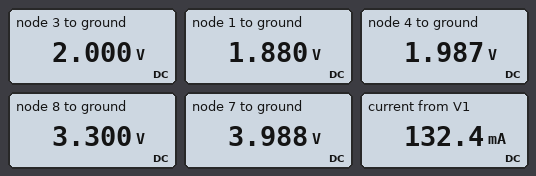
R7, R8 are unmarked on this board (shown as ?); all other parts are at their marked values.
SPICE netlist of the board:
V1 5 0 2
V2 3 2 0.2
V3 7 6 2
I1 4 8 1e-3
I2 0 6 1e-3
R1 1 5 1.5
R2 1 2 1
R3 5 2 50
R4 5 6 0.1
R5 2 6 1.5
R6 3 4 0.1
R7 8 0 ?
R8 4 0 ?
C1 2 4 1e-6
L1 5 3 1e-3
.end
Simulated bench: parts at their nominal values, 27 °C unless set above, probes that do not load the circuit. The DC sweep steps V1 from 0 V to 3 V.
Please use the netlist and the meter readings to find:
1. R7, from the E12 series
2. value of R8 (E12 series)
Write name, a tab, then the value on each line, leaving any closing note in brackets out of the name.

R7, from the E12 series	3.3 kΩ
value of R8	15 Ω
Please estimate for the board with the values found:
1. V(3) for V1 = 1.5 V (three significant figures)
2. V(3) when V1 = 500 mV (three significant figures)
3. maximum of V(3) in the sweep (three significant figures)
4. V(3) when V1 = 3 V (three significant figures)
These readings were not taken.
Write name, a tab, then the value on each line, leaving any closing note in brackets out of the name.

V(3) for V1 = 1.5 V	1.50 V
V(3) when V1 = 500 mV	500 mV
maximum of V(3) in the sweep	3.00 V
V(3) when V1 = 3 V	3.00 V
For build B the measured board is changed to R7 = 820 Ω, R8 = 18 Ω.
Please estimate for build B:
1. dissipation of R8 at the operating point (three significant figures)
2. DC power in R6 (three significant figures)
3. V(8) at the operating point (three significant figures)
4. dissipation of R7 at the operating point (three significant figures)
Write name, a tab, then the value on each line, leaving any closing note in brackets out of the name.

dissipation of R8 at the operating point	220 mW
DC power in R6	1.24 mW
V(8) at the operating point	820 mV
dissipation of R7 at the operating point	820 µW
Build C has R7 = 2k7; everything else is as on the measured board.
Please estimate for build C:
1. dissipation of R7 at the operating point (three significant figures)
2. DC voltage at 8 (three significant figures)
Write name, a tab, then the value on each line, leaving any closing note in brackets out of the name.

dissipation of R7 at the operating point	2.70 mW
DC voltage at 8	2.70 V
